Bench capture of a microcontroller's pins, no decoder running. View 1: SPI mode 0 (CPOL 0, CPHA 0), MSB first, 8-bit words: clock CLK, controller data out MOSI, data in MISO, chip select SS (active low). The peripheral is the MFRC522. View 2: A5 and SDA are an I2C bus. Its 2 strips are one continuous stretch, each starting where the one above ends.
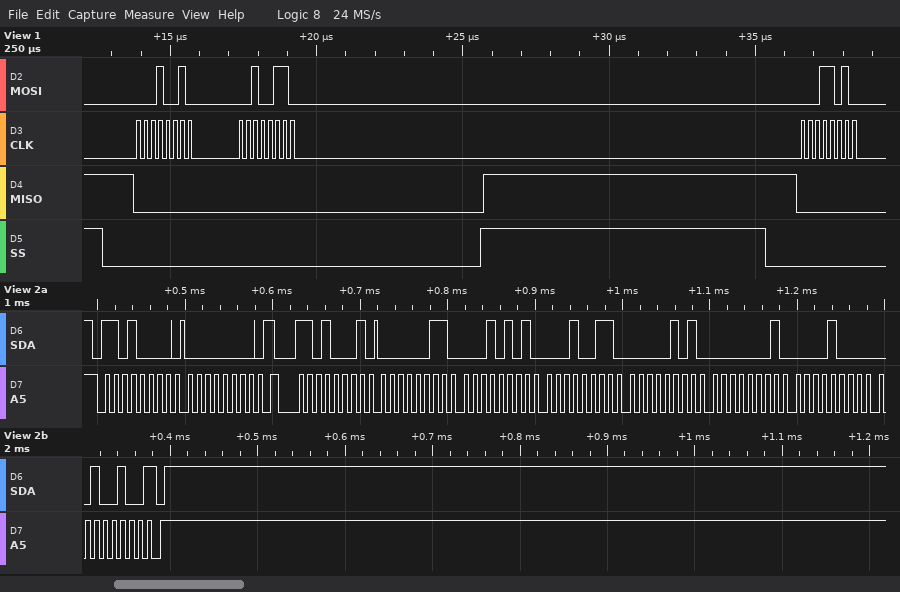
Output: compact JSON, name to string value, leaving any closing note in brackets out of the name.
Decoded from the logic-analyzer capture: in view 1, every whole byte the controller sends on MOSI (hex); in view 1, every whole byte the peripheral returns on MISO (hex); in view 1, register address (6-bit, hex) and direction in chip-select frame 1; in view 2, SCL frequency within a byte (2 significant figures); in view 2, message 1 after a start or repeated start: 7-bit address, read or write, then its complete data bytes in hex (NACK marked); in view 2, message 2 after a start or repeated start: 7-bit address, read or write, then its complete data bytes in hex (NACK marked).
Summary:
{"in view 1, every whole byte the controller sends on MOSI": "12 26 1A", "in view 1, every whole byte the peripheral returns on MISO": "00 00 00", "in view 1, register address (6-bit, hex) and direction in chip-select frame 1": "0x09 write", "in view 2, SCL frequency within a byte": "100 kHz", "in view 2, message 1 after a start or repeated start: 7-bit address, read or write, then its complete data bytes in hex": "0x68 write: 00", "in view 2, message 2 after a start or repeated start: 7-bit address, read or write, then its complete data bytes in hex": "0x68 read: 03 15 13 05 01 08 24 NACK"}
